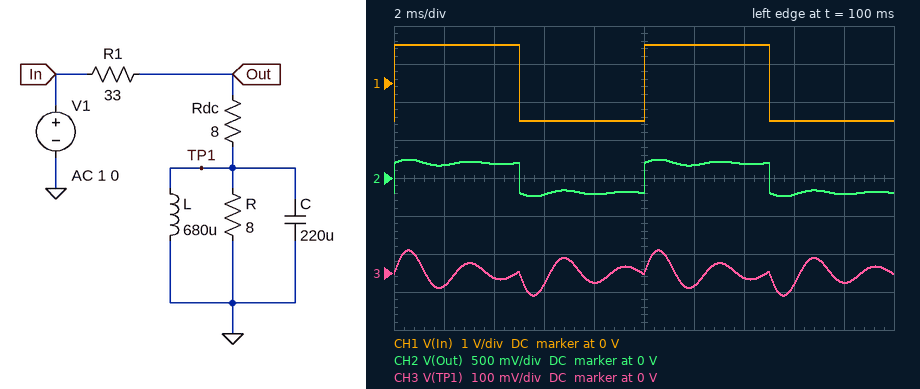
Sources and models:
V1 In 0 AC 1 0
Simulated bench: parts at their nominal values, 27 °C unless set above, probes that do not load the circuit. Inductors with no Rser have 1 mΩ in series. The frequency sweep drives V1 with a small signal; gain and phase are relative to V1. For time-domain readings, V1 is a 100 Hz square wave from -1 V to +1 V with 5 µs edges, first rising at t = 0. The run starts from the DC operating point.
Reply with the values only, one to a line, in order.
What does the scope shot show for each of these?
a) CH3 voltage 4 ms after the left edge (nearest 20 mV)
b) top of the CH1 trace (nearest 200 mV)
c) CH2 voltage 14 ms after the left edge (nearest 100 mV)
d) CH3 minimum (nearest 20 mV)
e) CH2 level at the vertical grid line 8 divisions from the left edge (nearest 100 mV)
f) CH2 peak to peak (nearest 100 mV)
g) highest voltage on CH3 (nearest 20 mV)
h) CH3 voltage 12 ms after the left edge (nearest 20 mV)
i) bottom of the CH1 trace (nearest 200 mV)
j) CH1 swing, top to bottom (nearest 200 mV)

-20 mV
1.0 V
200 mV
-60 mV
-200 mV
500 mV
60 mV
-40 mV
-1.0 V
2.0 V
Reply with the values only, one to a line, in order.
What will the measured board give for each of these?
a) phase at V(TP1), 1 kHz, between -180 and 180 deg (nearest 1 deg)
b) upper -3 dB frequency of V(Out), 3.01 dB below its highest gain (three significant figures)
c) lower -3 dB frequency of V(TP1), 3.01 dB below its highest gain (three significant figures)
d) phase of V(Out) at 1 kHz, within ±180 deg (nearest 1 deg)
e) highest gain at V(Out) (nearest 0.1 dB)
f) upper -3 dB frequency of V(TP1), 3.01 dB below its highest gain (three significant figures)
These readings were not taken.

-83 deg
525 Hz
361 Hz
-5 deg
-9.7 dB
469 Hz
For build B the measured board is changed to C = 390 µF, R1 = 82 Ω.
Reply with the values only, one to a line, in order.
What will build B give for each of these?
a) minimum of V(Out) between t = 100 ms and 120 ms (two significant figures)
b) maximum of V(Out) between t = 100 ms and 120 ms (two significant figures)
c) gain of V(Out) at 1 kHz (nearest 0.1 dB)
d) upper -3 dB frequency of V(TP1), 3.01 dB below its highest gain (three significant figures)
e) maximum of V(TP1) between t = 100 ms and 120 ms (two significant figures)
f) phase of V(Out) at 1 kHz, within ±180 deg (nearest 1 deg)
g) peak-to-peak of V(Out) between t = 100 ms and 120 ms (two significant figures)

-130 mV
130 mV
-21.0 dB
338 Hz
43 mV
-3 deg
260 mV
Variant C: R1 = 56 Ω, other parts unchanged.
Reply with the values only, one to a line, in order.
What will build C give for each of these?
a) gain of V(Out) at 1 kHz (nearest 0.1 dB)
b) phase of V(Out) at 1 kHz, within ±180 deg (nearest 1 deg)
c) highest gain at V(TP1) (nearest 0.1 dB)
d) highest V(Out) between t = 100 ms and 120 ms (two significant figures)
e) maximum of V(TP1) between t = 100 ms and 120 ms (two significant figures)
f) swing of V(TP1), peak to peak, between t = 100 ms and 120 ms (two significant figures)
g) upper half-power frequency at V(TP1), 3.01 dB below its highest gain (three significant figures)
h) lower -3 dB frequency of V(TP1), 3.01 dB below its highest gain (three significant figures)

-17.9 dB
-5 deg
-19.1 dB
160 mV
38 mV
76 mV
466 Hz
364 Hz
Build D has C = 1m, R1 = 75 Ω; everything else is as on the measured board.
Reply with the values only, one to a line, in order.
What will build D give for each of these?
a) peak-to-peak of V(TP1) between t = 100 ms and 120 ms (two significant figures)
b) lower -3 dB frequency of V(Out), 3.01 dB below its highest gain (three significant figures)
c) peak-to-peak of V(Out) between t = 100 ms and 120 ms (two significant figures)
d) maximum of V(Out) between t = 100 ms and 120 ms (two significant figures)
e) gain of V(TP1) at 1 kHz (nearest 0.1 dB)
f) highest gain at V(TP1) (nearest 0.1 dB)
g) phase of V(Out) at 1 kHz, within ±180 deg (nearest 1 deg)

22 mV
176 Hz
210 mV
110 mV
-54.0 dB
-21.2 dB
-1 deg
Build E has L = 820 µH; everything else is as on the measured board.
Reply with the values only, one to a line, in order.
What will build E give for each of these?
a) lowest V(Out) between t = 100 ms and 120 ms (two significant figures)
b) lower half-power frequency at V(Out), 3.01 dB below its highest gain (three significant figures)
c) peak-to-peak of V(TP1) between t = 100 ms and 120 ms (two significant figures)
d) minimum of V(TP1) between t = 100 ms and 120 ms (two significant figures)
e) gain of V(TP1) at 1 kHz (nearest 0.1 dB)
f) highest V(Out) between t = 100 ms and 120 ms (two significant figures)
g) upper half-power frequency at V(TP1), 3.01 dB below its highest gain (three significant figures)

-250 mV
287 Hz
140 mV
-70 mV
-33.8 dB
250 mV
433 Hz
